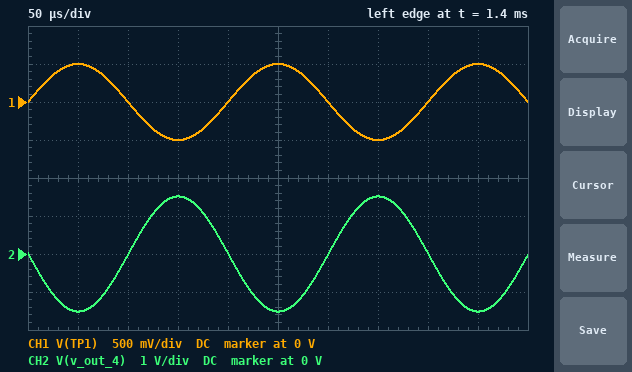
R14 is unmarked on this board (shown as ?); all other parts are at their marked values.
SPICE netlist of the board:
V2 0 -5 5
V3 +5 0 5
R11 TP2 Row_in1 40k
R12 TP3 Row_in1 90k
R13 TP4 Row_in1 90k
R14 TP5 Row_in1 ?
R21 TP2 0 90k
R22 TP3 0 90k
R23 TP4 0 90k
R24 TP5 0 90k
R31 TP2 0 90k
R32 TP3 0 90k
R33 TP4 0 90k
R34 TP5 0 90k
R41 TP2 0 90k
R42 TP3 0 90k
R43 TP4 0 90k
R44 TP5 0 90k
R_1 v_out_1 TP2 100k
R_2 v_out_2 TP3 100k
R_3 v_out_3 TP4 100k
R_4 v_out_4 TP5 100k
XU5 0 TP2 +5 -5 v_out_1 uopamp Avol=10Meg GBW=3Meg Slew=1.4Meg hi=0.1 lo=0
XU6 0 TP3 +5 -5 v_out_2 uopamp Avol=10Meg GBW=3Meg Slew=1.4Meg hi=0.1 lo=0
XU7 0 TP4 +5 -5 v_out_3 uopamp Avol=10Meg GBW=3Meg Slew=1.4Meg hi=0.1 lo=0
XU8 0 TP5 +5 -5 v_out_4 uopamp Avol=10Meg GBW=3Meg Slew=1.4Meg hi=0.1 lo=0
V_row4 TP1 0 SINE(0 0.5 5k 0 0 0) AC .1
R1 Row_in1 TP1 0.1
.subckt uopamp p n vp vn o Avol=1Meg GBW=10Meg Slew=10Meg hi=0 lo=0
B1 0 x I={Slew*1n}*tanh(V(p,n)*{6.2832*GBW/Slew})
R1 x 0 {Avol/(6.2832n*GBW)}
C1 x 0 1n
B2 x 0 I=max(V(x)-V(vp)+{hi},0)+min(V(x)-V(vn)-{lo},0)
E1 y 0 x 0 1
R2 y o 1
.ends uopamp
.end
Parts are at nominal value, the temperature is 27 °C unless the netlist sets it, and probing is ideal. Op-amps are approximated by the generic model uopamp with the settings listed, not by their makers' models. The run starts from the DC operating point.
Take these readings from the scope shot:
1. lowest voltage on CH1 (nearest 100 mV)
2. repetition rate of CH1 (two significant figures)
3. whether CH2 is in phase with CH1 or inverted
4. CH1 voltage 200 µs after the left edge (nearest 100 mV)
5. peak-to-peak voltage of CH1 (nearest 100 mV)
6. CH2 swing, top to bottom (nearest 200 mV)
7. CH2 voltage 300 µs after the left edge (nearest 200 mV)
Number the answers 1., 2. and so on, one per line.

1. -500 mV
2. 5.0 kHz
3. inverted
4. 0 V
5. 1.0 V
6. 3.0 V
7. 0 V
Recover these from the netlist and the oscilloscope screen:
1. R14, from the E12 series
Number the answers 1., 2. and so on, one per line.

1. 33 kΩ
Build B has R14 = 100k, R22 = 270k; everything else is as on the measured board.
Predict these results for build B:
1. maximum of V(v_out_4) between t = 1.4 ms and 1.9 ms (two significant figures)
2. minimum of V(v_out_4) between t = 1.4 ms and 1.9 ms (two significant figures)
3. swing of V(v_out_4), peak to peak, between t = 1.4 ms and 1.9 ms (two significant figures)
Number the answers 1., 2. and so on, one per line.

1. 500 mV
2. -500 mV
3. 1.0 V
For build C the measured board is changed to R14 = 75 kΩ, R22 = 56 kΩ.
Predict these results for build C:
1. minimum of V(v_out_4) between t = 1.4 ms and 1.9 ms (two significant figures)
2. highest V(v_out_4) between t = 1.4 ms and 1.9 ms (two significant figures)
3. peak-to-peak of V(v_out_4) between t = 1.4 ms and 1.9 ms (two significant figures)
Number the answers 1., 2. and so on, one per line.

1. -670 mV
2. 670 mV
3. 1.3 V
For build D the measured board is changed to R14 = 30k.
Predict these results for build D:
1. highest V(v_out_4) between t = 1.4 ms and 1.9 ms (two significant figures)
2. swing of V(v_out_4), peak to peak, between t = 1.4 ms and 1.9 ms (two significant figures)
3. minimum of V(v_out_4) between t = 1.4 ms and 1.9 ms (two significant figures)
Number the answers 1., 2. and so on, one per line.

1. 1.7 V
2. 3.3 V
3. -1.7 V
